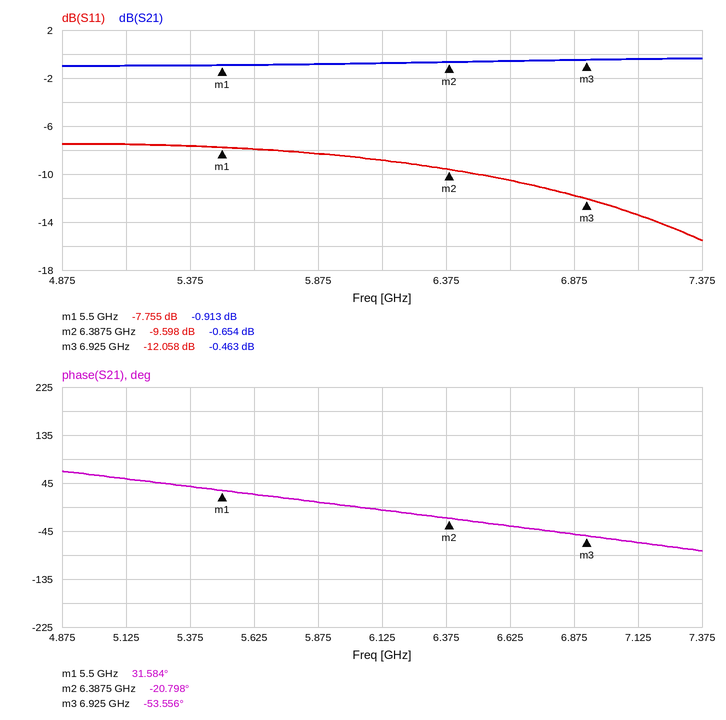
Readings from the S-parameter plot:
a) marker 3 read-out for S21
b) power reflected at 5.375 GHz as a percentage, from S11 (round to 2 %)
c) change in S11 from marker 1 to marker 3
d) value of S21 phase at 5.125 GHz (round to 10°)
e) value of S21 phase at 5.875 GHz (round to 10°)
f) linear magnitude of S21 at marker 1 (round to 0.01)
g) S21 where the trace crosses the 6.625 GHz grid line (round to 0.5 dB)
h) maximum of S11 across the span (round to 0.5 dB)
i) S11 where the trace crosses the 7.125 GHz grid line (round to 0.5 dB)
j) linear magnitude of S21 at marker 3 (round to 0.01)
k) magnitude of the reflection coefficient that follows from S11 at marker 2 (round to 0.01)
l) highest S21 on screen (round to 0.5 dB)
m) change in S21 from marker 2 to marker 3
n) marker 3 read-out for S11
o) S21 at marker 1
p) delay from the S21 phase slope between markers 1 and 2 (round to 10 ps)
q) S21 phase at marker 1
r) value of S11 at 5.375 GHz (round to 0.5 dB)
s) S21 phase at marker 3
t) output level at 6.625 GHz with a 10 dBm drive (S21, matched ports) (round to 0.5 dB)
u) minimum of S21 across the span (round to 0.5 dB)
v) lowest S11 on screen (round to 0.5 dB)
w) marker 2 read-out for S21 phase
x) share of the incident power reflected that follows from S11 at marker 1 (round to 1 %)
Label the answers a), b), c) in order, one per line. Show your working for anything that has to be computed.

a) -0.463 dB
b) 10^(-7.5/10) ≈ 18 %
c) -12.058 − (-7.755) = -4.303 dB
d) 50°
e) 10°
f) 10^(-0.913/20) ≈ 0.90
g) -0.5 dB
h) -7.5 dB
i) -13.5 dB
j) 10^(-0.463/20) ≈ 0.95
k) 10^(-9.598/20) ≈ 0.33
l) -0.5 dB
m) -0.463 − (-0.654) = 0.191 dB
n) -12.058 dB
o) -0.913 dB
p) −(-20.798° − (31.584°))/(360° × 887.5 MHz) ≈ 164 ps, so 160 ps to the nearest 10 ps
q) 31.584°
r) -7.5 dB
s) -53.556°
t) 10 dBm + (-0.5 dB) = 9.5 dBm
u) -1.0 dB
v) -15.5 dB
w) -20.798°
x) 10^(-7.755/10) ≈ 17 %
